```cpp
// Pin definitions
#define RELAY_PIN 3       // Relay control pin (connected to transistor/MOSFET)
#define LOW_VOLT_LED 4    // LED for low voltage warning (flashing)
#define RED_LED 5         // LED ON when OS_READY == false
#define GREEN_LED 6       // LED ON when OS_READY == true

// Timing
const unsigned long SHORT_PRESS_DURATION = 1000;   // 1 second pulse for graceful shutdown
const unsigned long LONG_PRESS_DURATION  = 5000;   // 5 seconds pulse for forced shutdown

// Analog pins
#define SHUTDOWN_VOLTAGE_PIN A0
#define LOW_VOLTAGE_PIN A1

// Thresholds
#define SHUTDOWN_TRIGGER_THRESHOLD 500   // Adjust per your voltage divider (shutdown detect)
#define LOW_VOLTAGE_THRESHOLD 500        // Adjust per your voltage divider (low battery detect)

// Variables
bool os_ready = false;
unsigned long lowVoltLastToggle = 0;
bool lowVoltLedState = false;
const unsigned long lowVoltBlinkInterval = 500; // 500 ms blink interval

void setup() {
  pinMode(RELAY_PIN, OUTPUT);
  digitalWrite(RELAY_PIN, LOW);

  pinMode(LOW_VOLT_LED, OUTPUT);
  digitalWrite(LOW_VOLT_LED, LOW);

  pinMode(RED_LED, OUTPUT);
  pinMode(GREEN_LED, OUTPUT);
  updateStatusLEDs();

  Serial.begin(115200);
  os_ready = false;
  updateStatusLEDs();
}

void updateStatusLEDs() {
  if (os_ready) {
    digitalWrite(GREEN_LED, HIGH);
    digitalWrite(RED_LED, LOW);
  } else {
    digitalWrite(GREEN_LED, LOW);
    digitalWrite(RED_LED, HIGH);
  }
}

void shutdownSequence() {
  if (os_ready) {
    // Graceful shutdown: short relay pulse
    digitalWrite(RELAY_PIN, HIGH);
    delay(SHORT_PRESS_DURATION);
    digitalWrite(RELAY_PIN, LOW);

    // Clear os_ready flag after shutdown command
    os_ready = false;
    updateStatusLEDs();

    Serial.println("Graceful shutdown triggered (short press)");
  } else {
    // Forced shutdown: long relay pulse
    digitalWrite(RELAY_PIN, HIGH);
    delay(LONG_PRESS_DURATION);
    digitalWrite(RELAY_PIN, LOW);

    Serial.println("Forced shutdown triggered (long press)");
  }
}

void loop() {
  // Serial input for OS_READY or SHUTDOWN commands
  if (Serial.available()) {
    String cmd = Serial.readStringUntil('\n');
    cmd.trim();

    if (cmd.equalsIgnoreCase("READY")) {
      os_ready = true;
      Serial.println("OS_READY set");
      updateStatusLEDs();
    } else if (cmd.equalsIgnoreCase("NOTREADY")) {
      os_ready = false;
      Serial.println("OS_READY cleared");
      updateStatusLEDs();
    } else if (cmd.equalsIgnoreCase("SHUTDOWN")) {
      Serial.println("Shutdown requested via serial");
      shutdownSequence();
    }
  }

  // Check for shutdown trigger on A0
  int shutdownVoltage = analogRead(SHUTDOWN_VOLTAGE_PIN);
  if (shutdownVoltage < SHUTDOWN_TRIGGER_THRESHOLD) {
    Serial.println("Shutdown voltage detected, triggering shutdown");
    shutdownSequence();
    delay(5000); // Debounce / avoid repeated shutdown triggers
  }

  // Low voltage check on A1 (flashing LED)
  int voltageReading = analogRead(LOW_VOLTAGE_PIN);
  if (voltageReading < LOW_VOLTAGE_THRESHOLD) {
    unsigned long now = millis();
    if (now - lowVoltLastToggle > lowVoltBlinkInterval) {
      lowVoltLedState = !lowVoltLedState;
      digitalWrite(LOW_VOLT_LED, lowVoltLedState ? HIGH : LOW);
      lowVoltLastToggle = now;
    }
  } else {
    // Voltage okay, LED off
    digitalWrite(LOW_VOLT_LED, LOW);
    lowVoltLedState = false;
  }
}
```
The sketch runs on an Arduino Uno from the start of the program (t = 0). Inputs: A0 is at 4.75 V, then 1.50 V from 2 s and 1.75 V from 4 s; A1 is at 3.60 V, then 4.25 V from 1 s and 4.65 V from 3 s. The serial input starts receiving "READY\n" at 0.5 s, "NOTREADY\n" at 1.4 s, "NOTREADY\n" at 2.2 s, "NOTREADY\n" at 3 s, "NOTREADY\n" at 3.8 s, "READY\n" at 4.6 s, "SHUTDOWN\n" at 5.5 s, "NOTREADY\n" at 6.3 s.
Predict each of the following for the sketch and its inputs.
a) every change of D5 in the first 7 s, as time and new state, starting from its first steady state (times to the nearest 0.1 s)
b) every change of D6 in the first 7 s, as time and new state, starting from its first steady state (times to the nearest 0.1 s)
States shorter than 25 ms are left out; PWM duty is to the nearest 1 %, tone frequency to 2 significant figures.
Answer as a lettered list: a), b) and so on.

a) 0 s high; 0.5 s low; 1.4 s high
b) 0 s low; 0.5 s high; 1.4 s low
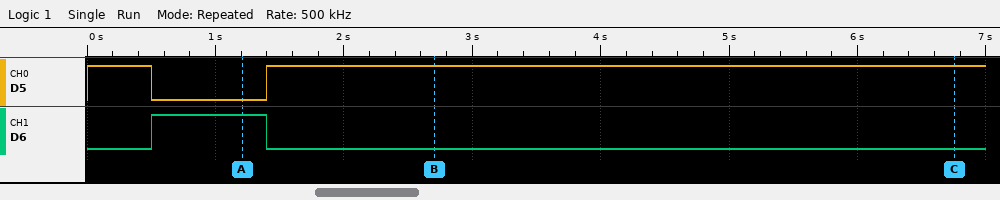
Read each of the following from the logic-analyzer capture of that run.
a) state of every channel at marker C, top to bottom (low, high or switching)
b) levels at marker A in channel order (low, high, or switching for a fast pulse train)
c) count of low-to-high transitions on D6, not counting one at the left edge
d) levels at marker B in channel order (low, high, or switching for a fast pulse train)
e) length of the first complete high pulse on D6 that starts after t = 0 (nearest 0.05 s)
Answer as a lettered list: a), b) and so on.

a) D5 high, D6 low
b) D5 low, D6 high
c) 1
d) D5 high, D6 low
e) 0.90 s
